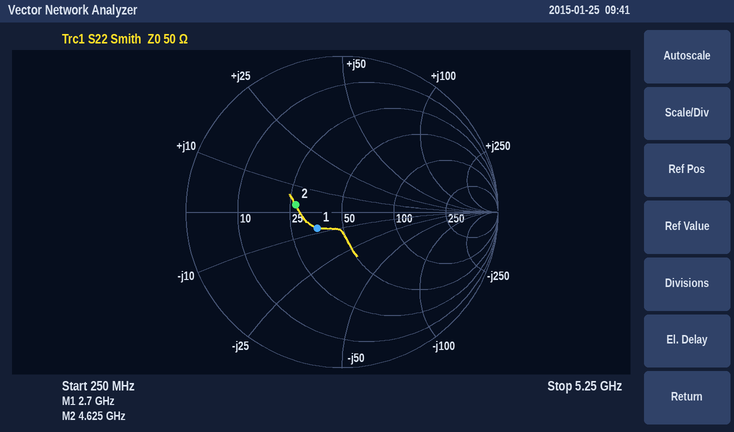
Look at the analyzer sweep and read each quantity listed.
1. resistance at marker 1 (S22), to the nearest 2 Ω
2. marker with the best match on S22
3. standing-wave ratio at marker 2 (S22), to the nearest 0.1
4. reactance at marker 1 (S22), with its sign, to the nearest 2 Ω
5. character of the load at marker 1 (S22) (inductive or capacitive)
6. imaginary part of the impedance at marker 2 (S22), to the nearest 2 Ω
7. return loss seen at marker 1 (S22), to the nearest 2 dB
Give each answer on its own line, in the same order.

36 Ω
marker 1
1.9
-8 Ω
capacitive
+2 Ω
14 dB
